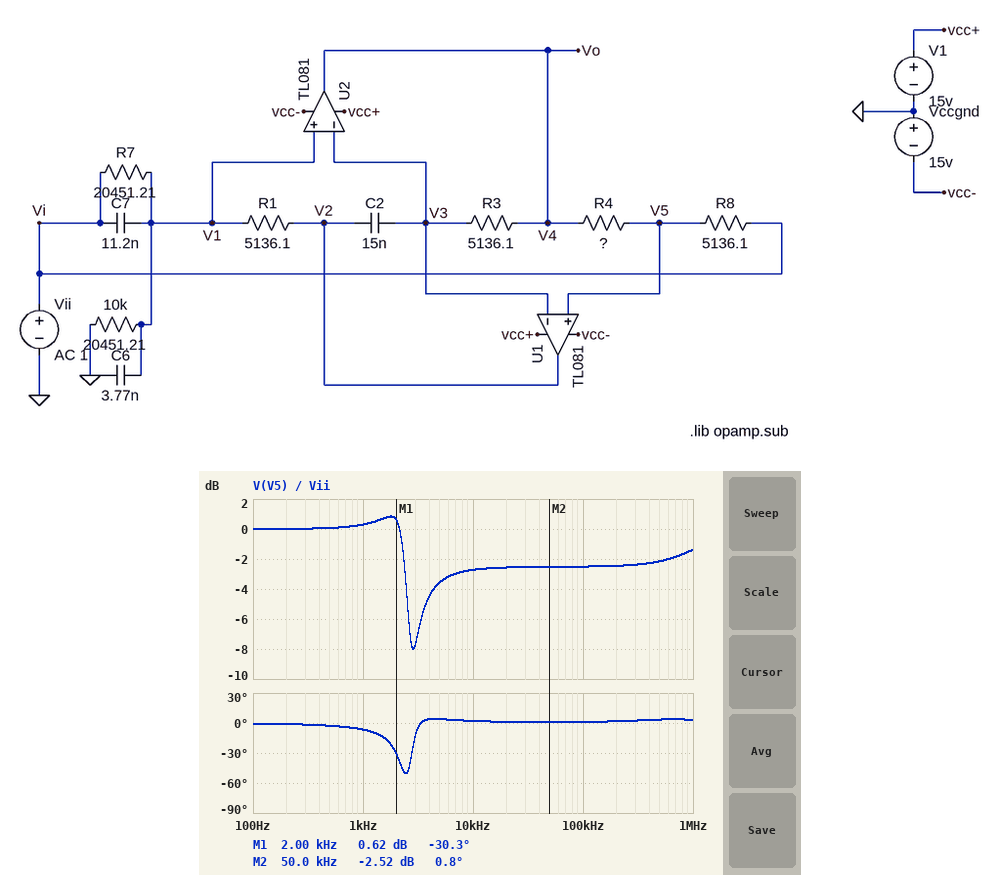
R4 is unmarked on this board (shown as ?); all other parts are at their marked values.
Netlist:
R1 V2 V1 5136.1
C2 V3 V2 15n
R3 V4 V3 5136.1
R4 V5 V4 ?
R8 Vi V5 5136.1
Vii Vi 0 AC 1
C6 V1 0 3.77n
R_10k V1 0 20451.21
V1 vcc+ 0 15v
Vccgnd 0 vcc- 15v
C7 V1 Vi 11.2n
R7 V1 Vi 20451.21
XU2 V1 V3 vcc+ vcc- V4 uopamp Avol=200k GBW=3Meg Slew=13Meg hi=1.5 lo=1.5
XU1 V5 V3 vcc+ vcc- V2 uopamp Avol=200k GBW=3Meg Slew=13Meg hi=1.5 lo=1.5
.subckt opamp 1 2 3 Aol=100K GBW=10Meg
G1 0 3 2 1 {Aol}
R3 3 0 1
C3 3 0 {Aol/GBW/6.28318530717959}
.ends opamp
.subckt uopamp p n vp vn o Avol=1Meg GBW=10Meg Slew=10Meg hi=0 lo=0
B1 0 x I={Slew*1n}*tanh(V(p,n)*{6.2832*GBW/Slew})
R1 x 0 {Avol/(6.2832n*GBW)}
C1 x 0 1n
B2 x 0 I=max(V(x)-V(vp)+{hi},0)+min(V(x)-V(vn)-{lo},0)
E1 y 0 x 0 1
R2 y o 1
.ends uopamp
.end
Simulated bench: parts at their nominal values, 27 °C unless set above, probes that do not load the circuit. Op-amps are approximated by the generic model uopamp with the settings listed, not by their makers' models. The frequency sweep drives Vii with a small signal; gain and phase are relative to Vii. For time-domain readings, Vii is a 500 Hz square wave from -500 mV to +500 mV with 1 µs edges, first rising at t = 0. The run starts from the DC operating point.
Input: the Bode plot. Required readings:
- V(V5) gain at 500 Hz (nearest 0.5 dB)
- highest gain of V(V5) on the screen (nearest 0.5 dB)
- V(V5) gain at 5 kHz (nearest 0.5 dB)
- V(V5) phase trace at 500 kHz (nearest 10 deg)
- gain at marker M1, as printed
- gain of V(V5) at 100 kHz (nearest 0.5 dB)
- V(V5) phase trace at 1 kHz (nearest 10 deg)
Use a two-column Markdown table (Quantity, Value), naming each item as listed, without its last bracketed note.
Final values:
| Quantity | Value |
|---|---|
| V(V5) gain at 500 Hz | 0 dB |
| highest gain of V(V5) on the screen | 1.0 dB |
| V(V5) gain at 5 kHz | -3.5 dB |
| V(V5) phase trace at 500 kHz | 0 deg |
| gain at marker M1, as printed | 0.62 dB |
| gain of V(V5) at 100 kHz | -2.5 dB |
| V(V5) phase trace at 1 kHz | -10 deg |
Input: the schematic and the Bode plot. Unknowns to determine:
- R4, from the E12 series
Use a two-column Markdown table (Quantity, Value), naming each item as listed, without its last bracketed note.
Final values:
| Quantity | Value |
|---|---|
| R4, from the E12 series | 6.8 kΩ |
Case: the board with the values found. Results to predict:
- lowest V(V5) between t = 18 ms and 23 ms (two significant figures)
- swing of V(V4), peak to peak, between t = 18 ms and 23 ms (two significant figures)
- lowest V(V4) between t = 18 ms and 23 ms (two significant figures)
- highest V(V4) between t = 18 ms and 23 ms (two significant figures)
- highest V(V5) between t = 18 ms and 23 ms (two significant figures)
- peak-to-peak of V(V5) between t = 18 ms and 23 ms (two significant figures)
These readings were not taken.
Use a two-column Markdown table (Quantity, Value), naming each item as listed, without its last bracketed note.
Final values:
| Quantity | Value |
|---|---|
| lowest V(V5) between t = 18 ms and 23 ms | -640 mV |
| swing of V(V4), peak to peak, between t = 18 ms and 23 ms | 1.6 V |
| lowest V(V4) between t = 18 ms and 23 ms | -820 mV |
| highest V(V4) between t = 18 ms and 23 ms | 820 mV |
| highest V(V5) between t = 18 ms and 23 ms | 640 mV |
| peak-to-peak of V(V5) between t = 18 ms and 23 ms | 1.3 V |
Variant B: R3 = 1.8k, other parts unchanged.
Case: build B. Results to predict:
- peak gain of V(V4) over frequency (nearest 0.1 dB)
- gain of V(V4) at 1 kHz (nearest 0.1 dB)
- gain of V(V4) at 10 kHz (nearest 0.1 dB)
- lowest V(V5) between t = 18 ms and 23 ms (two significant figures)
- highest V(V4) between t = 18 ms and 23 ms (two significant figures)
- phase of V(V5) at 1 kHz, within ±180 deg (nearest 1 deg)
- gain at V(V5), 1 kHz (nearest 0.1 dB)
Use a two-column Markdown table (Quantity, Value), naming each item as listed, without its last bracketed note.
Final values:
| Quantity | Value |
|---|---|
| peak gain of V(V4) over frequency | 7.5 dB |
| gain of V(V4) at 1 kHz | 0.3 dB |
| gain of V(V4) at 10 kHz | -10.4 dB |
| lowest V(V5) between t = 18 ms and 23 ms | -670 mV |
| highest V(V4) between t = 18 ms and 23 ms | 890 mV |
| phase of V(V5) at 1 kHz, within ±180 deg | -2 deg |
| gain at V(V5), 1 kHz | 0.1 dB |
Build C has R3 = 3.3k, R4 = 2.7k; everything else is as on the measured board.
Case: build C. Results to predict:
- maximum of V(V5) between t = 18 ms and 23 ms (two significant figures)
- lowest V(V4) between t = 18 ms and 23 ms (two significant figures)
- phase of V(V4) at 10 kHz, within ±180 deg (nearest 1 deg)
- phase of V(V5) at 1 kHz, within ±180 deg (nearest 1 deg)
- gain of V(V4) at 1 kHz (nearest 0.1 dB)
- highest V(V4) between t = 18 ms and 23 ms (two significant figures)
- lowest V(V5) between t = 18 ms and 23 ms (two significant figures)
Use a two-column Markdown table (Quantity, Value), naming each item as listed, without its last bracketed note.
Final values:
| Quantity | Value |
|---|---|
| maximum of V(V5) between t = 18 ms and 23 ms | 610 mV |
| lowest V(V4) between t = 18 ms and 23 ms | -670 mV |
| phase of V(V4) at 10 kHz, within ±180 deg | 4 deg |
| phase of V(V5) at 1 kHz, within ±180 deg | -12 deg |
| gain of V(V4) at 1 kHz | 0.6 dB |
| highest V(V4) between t = 18 ms and 23 ms | 670 mV |
| lowest V(V5) between t = 18 ms and 23 ms | -610 mV |
